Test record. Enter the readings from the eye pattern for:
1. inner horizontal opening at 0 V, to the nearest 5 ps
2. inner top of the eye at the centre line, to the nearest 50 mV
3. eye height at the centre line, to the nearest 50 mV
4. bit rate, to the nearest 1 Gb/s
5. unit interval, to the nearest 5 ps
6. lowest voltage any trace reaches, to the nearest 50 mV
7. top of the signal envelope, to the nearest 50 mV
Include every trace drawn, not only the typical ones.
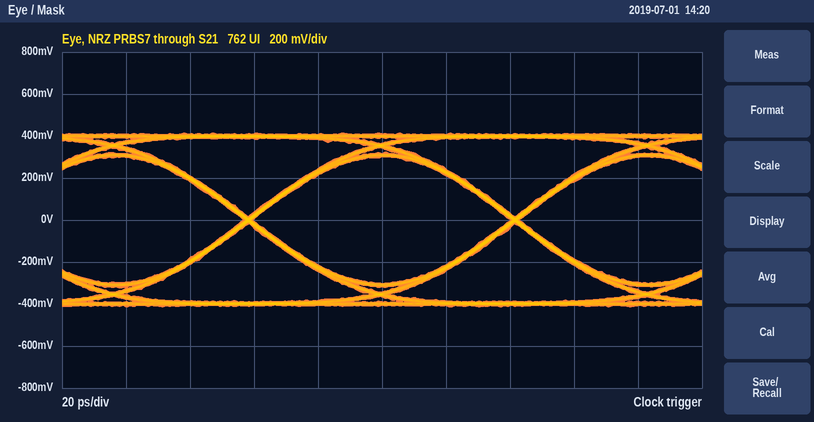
80 ps
300 mV
600 mV
12 Gb/s
85 ps
-400 mV
400 mV
